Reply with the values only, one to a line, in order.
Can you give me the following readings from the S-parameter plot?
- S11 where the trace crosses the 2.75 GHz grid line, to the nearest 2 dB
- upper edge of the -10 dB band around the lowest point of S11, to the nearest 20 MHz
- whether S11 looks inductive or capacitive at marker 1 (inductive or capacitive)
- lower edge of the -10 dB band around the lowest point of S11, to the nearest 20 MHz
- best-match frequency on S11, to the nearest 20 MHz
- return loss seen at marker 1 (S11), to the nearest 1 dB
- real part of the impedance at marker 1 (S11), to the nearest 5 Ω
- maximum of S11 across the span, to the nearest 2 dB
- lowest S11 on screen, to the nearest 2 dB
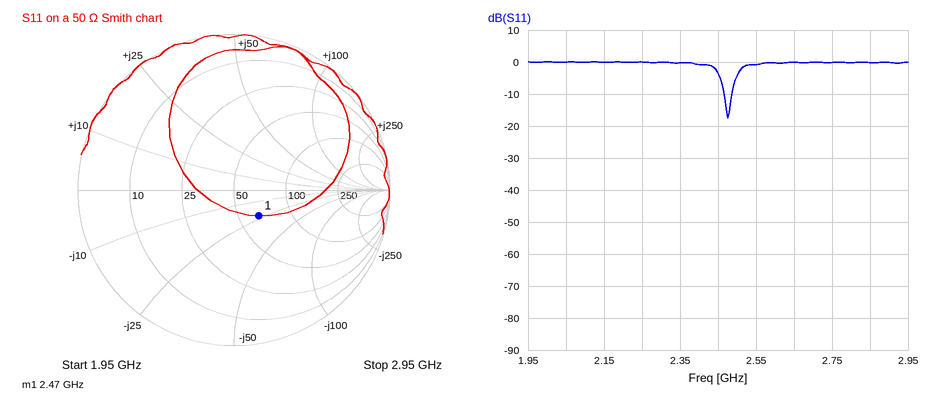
0 dB
2.48 GHz
capacitive
2.46 GHz
2.48 GHz
13 dB
65 Ω
0 dB
-18 dB
